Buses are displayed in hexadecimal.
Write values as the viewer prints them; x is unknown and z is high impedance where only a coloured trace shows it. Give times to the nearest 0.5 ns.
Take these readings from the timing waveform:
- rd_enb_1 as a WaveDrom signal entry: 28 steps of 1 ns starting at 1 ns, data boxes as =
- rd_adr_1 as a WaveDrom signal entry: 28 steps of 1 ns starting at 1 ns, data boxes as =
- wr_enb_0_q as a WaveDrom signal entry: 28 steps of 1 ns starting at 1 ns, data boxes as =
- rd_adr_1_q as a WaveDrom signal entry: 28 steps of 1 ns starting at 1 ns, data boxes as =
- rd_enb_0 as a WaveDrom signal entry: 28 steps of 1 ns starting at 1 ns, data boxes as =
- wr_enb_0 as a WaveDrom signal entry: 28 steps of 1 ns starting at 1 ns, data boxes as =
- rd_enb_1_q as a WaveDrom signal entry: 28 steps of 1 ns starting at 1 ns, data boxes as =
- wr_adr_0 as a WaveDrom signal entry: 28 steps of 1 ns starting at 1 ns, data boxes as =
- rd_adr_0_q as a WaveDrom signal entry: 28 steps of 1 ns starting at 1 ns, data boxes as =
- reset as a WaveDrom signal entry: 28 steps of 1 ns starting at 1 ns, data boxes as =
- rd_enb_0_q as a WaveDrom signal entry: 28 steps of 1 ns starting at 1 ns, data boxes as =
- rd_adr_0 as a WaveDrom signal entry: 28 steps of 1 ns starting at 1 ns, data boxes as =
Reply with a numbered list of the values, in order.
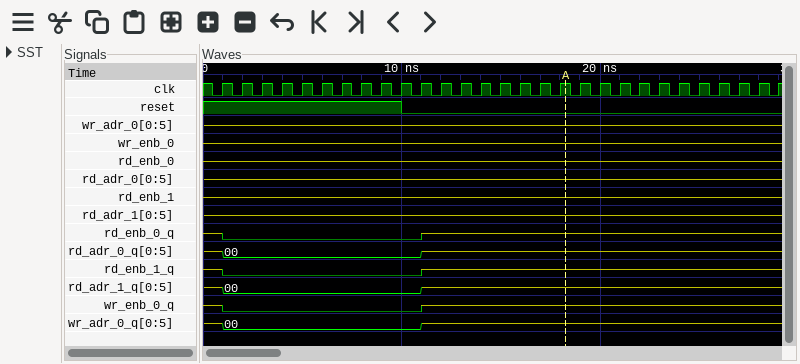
1. {name: 'rd_enb_1', wave: 'z...........................'}
2. {name: 'rd_adr_1', wave: 'z...........................'}
3. {name: 'wr_enb_0_q', wave: '0.........z.................'}
4. {name: 'rd_adr_1_q', wave: '=.........z.................', data: '00'}
5. {name: 'rd_enb_0', wave: 'z...........................'}
6. {name: 'wr_enb_0', wave: 'z...........................'}
7. {name: 'rd_enb_1_q', wave: '0.........z.................'}
8. {name: 'wr_adr_0', wave: 'z...........................'}
9. {name: 'rd_adr_0_q', wave: '=.........z.................', data: '00'}
10. {name: 'reset', wave: '1........0..................'}
11. {name: 'rd_enb_0_q', wave: '0.........z.................'}
12. {name: 'rd_adr_0', wave: 'z...........................'}
